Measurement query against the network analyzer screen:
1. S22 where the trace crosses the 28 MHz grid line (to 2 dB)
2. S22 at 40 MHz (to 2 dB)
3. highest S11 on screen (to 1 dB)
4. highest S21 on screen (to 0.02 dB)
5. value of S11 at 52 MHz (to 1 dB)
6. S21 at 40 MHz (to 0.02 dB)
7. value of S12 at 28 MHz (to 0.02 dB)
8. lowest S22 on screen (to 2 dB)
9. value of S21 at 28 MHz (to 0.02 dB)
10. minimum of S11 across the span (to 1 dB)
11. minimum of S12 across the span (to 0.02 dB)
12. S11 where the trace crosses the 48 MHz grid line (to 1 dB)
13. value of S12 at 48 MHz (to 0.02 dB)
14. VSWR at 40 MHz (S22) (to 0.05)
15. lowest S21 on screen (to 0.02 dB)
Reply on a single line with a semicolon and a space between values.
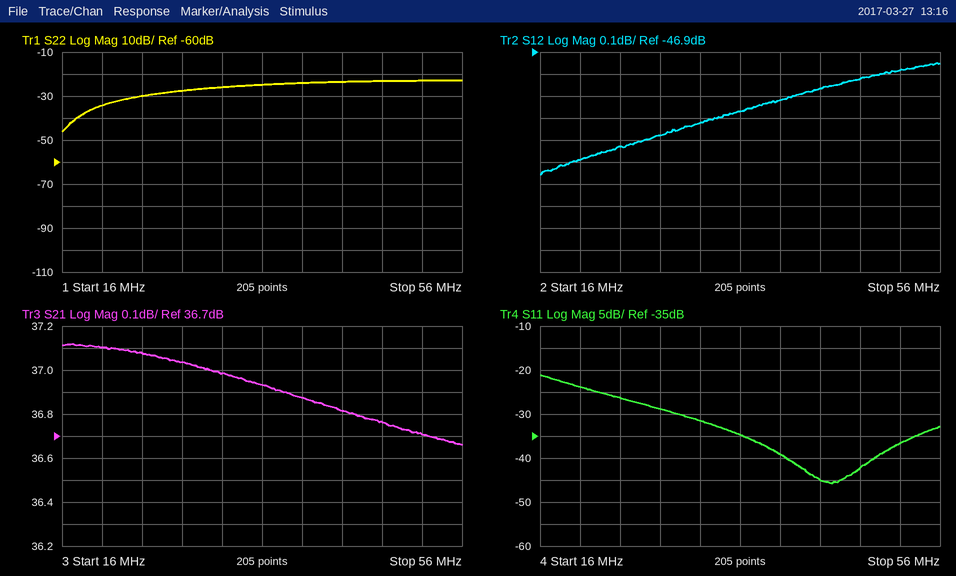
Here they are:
-28 dB; -24 dB; -21 dB; 37.12 dB; -37 dB; 36.88 dB; -47.28 dB; -46 dB; 37.04 dB; -46 dB; -47.46 dB; -42 dB; -47.02 dB; 1.15; 36.66 dB
